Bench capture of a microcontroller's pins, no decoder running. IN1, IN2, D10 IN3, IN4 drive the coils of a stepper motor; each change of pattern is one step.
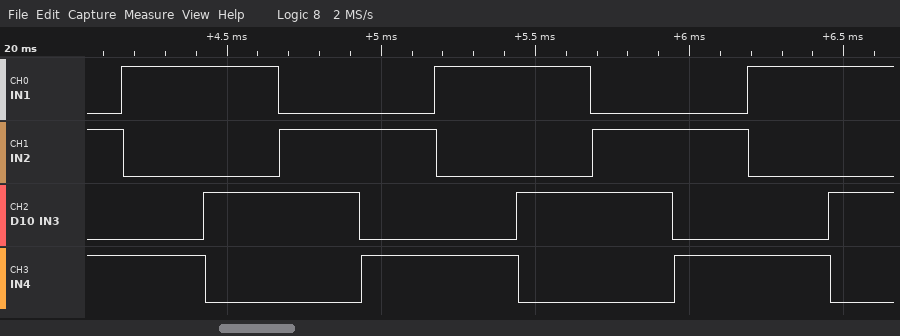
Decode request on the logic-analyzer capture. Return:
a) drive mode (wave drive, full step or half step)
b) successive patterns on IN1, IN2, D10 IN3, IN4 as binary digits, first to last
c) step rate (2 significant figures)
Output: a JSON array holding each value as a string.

["full step", "0101 1001 1010 0110 0101 1001 1010 0110 0101 1001 1010", "3900 steps/s"]
